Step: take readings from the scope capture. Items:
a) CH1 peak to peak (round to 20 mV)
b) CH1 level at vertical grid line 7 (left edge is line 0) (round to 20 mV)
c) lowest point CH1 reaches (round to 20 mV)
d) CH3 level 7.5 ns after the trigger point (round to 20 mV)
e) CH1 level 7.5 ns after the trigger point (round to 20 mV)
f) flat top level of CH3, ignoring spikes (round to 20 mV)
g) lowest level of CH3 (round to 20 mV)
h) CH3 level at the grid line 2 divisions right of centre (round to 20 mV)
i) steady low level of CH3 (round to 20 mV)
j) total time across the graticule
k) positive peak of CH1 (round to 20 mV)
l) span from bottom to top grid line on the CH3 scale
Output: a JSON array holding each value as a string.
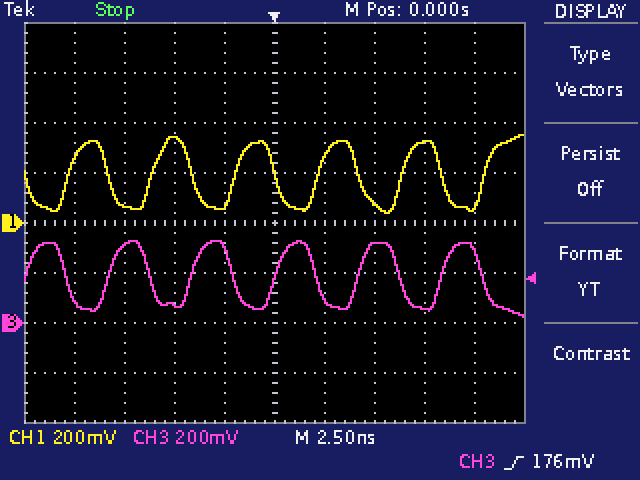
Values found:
["320 mV", "80 mV", "40 mV", "60 mV", "320 mV", "320 mV", "20 mV", "320 mV", "60 mV", "25 ns", "360 mV", "1.6 V"]
